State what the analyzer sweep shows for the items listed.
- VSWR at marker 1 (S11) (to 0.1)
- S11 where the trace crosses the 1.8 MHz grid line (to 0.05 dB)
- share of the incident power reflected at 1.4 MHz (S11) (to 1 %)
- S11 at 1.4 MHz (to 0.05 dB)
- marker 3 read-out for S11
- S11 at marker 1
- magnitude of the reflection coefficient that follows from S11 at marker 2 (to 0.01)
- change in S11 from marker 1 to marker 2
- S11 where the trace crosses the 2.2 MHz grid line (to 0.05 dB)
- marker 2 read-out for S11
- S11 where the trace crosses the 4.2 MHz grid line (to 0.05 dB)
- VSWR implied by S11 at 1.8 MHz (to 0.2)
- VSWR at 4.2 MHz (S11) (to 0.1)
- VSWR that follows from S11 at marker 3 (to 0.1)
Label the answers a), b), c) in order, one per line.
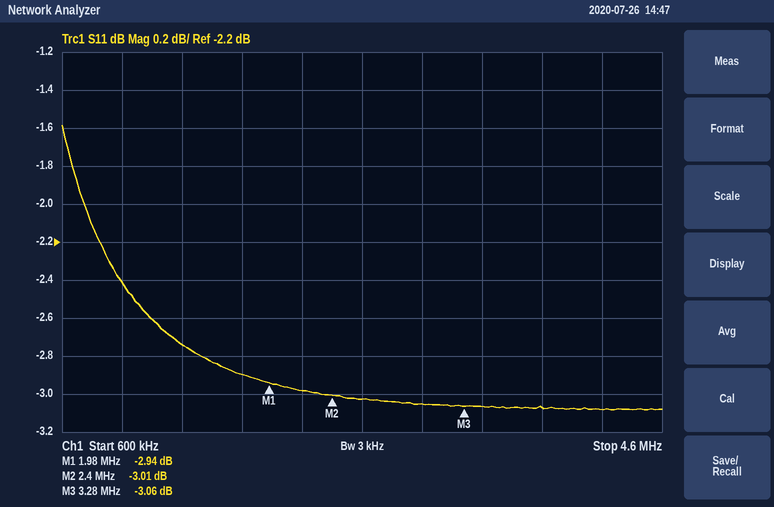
a) 6.0
b) -2.90 dB
c) 53 %
d) -2.75 dB
e) -3.06 dB
f) -2.94 dB
g) 0.71
h) -0.07 dB
i) -3.00 dB
j) -3.01 dB
k) -3.10 dB
l) 6.0
m) 5.7
n) 5.7
